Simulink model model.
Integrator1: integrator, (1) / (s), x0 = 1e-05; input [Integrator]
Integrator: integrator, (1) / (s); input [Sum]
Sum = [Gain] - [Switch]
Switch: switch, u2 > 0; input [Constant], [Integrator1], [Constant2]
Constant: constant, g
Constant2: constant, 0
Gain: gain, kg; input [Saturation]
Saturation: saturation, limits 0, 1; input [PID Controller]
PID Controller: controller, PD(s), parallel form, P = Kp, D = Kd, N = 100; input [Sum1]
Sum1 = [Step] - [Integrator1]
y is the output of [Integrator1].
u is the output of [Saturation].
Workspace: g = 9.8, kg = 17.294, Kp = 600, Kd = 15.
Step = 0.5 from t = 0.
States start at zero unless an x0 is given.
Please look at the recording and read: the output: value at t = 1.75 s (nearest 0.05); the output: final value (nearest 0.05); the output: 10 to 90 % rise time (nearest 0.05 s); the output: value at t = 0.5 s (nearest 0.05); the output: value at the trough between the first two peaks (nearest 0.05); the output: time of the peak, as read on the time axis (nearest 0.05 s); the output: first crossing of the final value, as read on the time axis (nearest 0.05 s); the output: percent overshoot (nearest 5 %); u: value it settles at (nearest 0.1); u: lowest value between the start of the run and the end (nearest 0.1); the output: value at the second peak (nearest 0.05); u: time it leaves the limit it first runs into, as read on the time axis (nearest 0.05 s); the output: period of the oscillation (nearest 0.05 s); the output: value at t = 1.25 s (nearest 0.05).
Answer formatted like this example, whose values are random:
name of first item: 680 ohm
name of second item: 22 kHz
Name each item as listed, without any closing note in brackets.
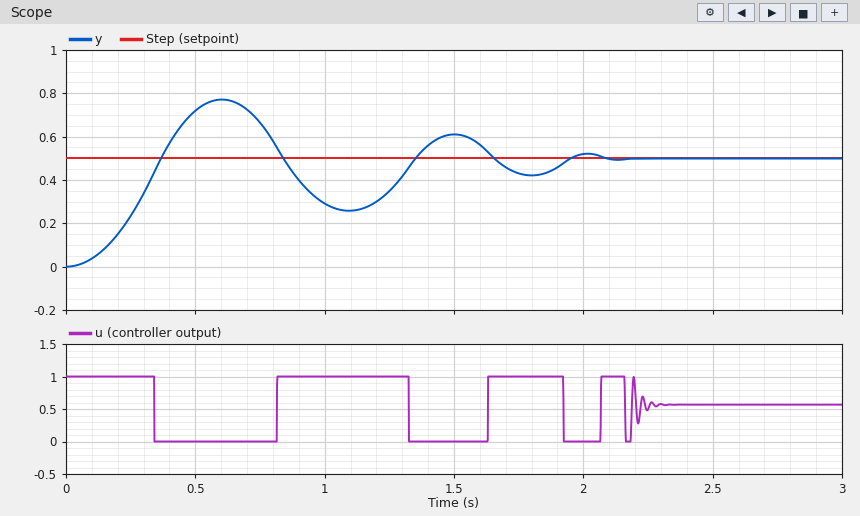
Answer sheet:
the output: value at t = 1.75 s: 0.45
the output: final value: 0.50
the output: 10 to 90 % rise time: 0.25 s
the output: value at t = 0.5 s: 0.70
the output: value at the trough between the first two peaks: 0.25
the output: time of the peak, as read on the time axis: 0.60 s
the output: first crossing of the final value, as read on the time axis: 0.35 s
the output: percent overshoot: 55 %
u: value it settles at: 0.6
u: lowest value between the start of the run and the end: 0.0
the output: value at the second peak: 0.60
u: time it leaves the limit it first runs into, as read on the time axis: 0.35 s
the output: period of the oscillation: 0.90 s
the output: value at t = 1.25 s: 0.35
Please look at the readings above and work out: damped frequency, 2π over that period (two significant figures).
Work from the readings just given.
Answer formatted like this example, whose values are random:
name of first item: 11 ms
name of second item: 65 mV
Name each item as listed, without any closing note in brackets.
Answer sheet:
damped frequency, 2π over that period: 7.0 rad/s
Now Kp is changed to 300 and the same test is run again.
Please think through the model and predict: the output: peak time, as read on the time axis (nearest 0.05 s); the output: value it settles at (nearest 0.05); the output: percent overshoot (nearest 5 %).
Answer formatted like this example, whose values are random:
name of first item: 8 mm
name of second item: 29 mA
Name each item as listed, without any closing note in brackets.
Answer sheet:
the output: peak time, as read on the time axis: 0.55 s
the output: value it settles at: 0.50
the output: percent overshoot: 35 %
